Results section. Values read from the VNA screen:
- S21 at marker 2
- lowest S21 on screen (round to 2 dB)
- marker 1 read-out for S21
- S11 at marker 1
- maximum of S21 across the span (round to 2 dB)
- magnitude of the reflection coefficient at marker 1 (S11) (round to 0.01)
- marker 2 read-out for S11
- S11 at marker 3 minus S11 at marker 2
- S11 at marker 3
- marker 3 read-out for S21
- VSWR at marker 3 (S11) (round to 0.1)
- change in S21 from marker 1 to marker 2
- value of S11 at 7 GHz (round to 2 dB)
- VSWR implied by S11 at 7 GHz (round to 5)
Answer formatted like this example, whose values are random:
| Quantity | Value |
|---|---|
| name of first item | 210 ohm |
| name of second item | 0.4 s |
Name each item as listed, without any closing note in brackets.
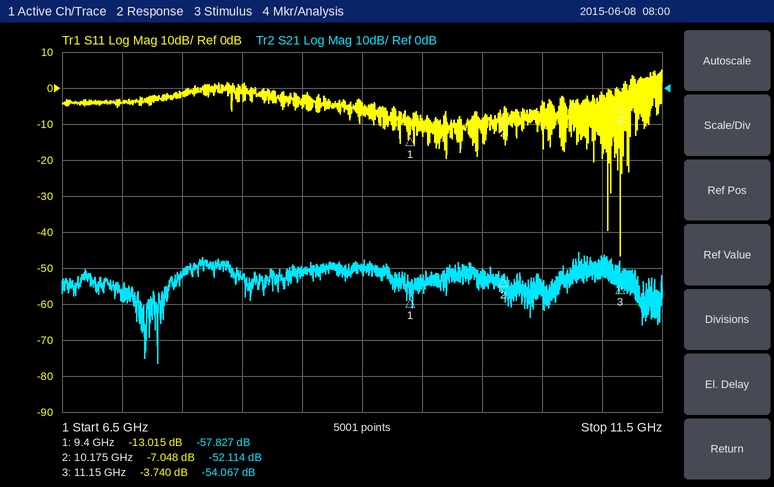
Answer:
| Quantity | Value |
|---|---|
| S21 at marker 2 | -52.114 dB |
| lowest S21 on screen | -76 dB |
| marker 1 read-out for S21 | -57.827 dB |
| S11 at marker 1 | -13.015 dB |
| maximum of S21 across the span | -46 dB |
| magnitude of the reflection coefficient at marker 1 (S11) | 0.22 |
| marker 2 read-out for S11 | -7.048 dB |
| S11 at marker 3 minus S11 at marker 2 | 3.308 dB |
| S11 at marker 3 | -3.740 dB |
| marker 3 read-out for S21 | -54.067 dB |
| VSWR at marker 3 (S11) | 4.7 |
| change in S21 from marker 1 to marker 2 | 5.713 dB |
| value of S11 at 7 GHz | -4 dB |
| VSWR implied by S11 at 7 GHz | 5 |
